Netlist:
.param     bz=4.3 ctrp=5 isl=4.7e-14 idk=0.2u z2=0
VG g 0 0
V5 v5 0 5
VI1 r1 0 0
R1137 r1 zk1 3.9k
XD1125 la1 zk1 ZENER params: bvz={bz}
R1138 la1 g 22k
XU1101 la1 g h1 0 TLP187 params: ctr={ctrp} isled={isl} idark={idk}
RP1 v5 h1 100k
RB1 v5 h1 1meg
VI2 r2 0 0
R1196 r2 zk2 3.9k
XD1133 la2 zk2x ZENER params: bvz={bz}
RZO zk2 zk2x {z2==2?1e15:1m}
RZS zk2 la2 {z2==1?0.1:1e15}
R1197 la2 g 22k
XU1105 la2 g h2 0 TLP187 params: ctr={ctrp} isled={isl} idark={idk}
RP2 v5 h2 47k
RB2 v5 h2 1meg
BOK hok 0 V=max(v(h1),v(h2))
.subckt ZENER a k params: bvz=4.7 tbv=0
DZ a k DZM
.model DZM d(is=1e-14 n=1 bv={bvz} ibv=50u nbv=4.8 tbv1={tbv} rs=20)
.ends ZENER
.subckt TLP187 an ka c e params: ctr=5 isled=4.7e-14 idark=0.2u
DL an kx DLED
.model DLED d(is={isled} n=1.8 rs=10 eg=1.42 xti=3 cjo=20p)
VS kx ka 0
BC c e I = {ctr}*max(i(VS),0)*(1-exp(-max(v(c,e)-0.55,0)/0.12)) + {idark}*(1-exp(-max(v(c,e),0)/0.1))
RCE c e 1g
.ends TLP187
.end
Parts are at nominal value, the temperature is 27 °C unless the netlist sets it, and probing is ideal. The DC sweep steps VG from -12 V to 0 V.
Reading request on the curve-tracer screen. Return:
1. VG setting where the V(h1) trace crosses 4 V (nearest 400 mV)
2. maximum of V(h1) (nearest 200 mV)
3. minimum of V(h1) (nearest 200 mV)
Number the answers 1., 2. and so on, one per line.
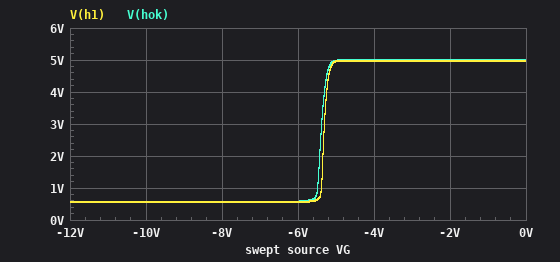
1. -5.2 V
2. 5.0 V
3. 600 mV
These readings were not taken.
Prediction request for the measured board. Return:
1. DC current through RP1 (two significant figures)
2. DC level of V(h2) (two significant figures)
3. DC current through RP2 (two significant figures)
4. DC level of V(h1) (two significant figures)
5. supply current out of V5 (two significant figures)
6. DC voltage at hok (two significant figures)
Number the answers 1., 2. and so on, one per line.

1. 190 nA
2. 5.0 V
3. 200 nA
4. 5.0 V
5. 410 nA
6. 5.0 V
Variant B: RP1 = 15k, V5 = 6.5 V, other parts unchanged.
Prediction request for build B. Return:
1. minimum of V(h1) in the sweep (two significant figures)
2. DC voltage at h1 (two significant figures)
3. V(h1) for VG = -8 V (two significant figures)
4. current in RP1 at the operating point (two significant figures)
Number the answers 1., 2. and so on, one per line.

1. 560 mV
2. 6.5 V
3. 570 mV
4. 200 nA
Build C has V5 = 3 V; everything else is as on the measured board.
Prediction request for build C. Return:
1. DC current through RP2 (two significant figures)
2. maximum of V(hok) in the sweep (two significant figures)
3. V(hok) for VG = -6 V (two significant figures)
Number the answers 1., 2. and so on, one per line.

1. 190 nA
2. 3.0 V
3. 560 mV
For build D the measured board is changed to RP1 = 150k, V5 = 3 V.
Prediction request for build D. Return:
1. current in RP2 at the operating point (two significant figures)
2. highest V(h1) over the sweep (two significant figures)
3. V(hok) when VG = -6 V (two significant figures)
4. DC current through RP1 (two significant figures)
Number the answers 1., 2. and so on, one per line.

1. 190 nA
2. 3.0 V
3. 560 mV
4. 180 nA
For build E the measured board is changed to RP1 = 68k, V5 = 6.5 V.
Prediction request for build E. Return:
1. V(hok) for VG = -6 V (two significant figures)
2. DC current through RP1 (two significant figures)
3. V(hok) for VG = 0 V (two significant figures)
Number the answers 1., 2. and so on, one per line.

1. 590 mV
2. 190 nA
3. 6.5 V
